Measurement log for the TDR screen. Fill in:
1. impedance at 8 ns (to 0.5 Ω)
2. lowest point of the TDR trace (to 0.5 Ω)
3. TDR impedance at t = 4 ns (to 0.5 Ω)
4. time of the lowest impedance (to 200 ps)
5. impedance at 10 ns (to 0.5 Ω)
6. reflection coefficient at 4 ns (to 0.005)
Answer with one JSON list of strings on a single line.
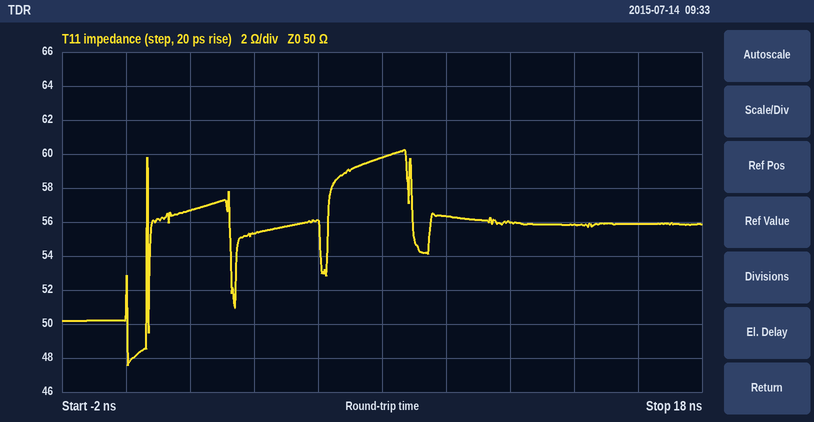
["60.0 Ω", "47.5 Ω", "55.5 Ω", "0.0 ns", "56.5 Ω", "+0.050"]
